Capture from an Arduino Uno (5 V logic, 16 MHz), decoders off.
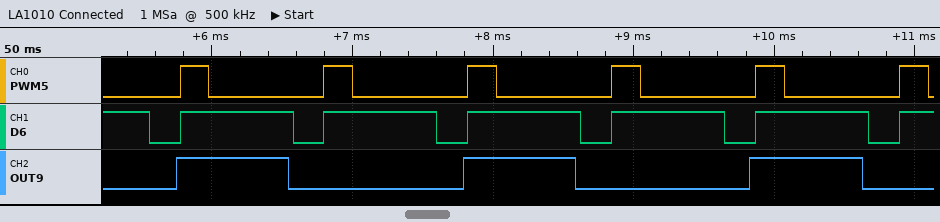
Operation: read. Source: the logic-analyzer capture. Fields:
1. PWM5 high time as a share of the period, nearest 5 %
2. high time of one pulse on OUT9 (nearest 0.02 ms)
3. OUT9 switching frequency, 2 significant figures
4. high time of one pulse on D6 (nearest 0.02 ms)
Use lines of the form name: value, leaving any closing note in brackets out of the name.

PWM5 high time as a share of the period, nearest 5 %: 20 %
high time of one pulse on OUT9: 0.80 ms
OUT9 switching frequency, 2 significant figures: 490 Hz
high time of one pulse on D6: 0.80 ms
